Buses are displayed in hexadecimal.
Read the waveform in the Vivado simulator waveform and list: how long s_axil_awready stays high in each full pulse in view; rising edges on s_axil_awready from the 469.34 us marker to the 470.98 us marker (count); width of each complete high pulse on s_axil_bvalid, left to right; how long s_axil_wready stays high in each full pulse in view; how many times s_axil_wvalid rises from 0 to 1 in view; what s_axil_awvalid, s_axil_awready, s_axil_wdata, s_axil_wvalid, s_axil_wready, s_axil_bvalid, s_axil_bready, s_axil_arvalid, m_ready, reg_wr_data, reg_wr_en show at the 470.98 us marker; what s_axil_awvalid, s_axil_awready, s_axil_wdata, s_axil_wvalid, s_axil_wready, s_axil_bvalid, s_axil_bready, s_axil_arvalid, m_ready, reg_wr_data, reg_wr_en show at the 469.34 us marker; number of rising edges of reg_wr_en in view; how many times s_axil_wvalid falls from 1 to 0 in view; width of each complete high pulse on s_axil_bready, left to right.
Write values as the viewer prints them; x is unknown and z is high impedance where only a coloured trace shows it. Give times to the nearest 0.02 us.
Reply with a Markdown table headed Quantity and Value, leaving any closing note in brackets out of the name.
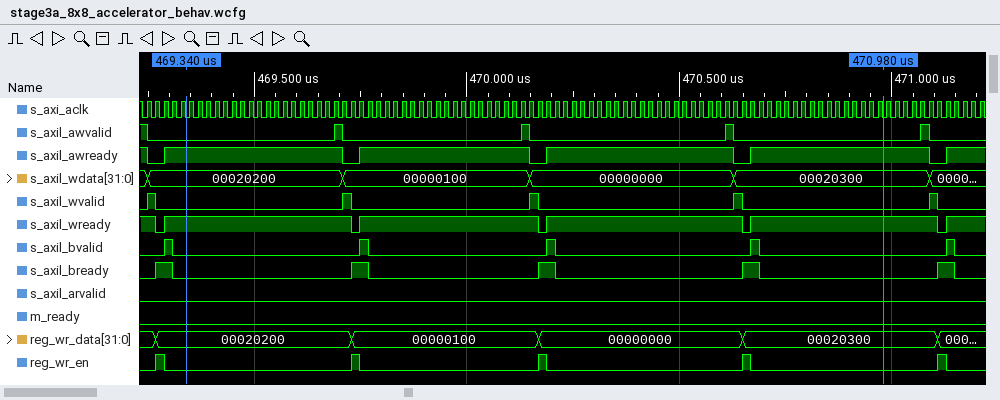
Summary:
| Quantity | Value |
|---|---|
| how long s_axil_awready stays high in each full pulse in view | 0.42 us, 0.4 us, 0.44 us, 0.42 us |
| rising edges on s_axil_awready from the 469.34 us marker to the 470.98 us marker | 3 |
| width of each complete high pulse on s_axil_bvalid, left to right | 0.02 us, 0.02 us, 0.02 us, 0.02 us, 0.02 us |
| how long s_axil_wready stays high in each full pulse in view | 0.44 us, 0.42 us, 0.46 us, 0.44 us |
| how many times s_axil_wvalid rises from 0 to 1 in view | 5 |
| what s_axil_awvalid, s_axil_awready, s_axil_wdata, s_axil_wvalid, s_axil_wready, s_axil_bvalid, s_axil_bready, s_axil_arvalid, m_ready, reg_wr_data, reg_wr_en show at the 470.98 us marker | s_axil_awvalid=0, s_axil_awready=1, s_axil_wdata=00020300, s_axil_wvalid=0, s_axil_wready=1, s_axil_bvalid=0, s_axil_bready=0, s_axil_arvalid=0, m_ready=0, reg_wr_data=00020300, reg_wr_en=0 |
| what s_axil_awvalid, s_axil_awready, s_axil_wdata, s_axil_wvalid, s_axil_wready, s_axil_bvalid, s_axil_bready, s_axil_arvalid, m_ready, reg_wr_data, reg_wr_en show at the 469.34 us marker | s_axil_awvalid=0, s_axil_awready=1, s_axil_wdata=00020200, s_axil_wvalid=0, s_axil_wready=1, s_axil_bvalid=0, s_axil_bready=0, s_axil_arvalid=0, m_ready=0, reg_wr_data=00020200, reg_wr_en=0 |
| number of rising edges of reg_wr_en in view | 5 |
| how many times s_axil_wvalid falls from 1 to 0 in view | 5 |
| width of each complete high pulse on s_axil_bready, left to right | 0.04 us, 0.04 us, 0.04 us, 0.04 us, 0.04 us |
